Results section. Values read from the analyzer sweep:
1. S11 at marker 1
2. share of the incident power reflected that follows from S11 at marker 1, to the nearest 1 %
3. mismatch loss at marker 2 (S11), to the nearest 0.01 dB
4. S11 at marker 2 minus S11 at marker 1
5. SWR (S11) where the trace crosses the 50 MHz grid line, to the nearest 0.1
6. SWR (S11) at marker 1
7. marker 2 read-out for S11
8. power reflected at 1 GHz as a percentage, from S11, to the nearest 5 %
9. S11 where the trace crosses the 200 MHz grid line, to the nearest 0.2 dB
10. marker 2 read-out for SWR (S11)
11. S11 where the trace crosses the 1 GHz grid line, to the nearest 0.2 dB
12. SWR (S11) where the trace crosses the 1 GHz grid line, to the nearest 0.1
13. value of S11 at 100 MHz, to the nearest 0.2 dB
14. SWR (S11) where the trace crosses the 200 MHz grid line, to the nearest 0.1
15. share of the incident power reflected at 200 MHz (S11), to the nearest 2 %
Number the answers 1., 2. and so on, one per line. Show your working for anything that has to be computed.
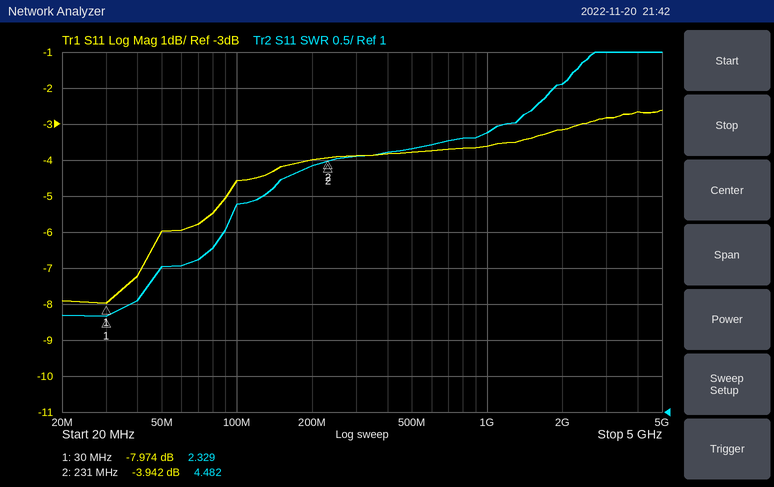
1. -7.974 dB
2. 10^(-7.974/10) ≈ 16 %
3. −10 log10(1 − 10^(-3.942/10)) ≈ 2.24 dB
4. -3.942 − (-7.974) = 4.032 dB
5. 3.0
6. 2.329
7. -3.942 dB
8. 10^(-3.6/10) ≈ 43.7 %, so 45 % to the nearest 5 %
9. -4.0 dB
10. 4.482
11. -3.6 dB
12. 4.9
13. -4.6 dB
14. 4.4
15. 10^(-4/10) ≈ 40 %
